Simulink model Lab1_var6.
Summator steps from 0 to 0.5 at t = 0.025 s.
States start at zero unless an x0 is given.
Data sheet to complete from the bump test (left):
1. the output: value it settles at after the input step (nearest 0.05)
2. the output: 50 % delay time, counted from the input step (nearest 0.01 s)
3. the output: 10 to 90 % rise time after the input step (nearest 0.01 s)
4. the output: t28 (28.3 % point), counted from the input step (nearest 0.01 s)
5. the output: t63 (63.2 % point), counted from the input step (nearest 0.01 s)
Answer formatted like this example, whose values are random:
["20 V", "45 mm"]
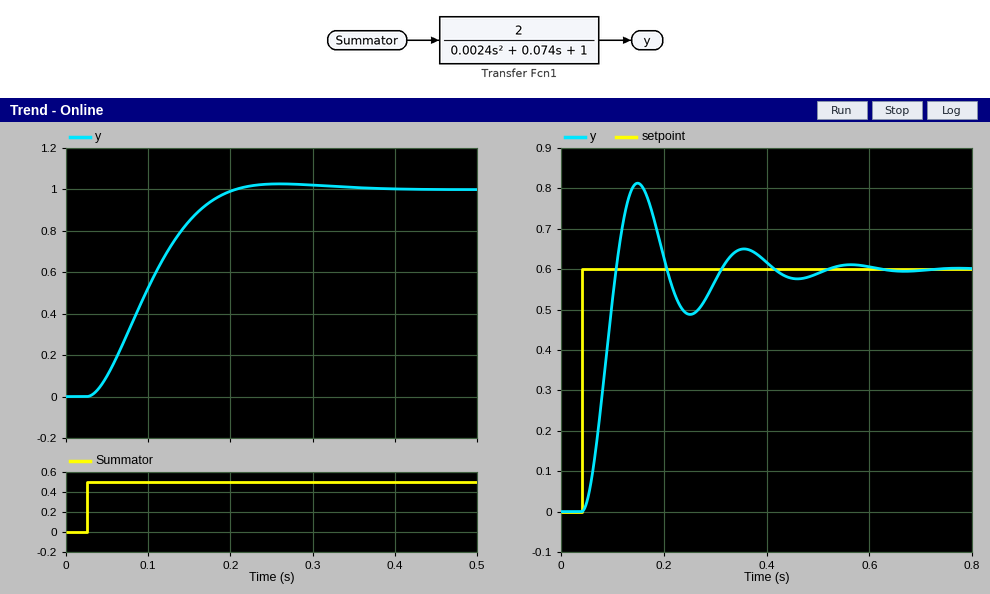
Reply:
["1.00", "0.07 s", "0.11 s", "0.05 s", "0.09 s"]
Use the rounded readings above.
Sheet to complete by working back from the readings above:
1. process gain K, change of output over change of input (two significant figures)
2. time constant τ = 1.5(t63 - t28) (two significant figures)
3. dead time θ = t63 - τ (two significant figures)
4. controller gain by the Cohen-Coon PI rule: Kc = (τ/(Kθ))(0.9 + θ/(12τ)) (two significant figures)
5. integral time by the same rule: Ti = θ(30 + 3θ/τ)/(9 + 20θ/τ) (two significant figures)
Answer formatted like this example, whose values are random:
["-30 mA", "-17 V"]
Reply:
["2.0", "0.060 s", "0.030 s", "0.94", "0.050 s"]
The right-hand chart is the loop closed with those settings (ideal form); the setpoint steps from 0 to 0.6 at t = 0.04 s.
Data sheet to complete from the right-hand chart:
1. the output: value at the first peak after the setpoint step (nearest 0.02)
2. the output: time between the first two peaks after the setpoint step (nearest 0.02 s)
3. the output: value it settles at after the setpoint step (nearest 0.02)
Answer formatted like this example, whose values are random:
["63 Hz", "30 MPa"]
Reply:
["0.82", "0.20 s", "0.60"]
